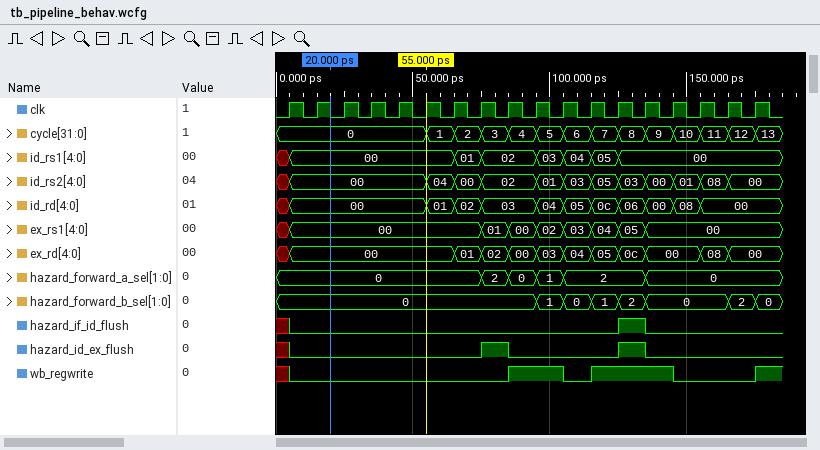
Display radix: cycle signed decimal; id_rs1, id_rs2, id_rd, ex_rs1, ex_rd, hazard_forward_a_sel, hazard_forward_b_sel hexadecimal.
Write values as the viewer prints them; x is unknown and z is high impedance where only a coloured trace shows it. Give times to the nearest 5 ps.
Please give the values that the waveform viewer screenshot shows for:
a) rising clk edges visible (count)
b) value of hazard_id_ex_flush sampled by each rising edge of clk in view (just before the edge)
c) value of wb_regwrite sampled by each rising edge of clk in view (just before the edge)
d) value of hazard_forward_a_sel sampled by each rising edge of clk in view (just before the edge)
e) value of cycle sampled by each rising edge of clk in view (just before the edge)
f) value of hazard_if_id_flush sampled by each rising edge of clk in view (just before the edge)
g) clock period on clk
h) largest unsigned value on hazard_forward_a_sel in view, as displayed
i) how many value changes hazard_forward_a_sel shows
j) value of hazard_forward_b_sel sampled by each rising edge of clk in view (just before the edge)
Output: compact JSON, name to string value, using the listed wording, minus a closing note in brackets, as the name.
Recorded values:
{"rising clk edges visible": "18", "value of hazard_id_ex_flush sampled by each rising edge of clk in view": "x 0 0 0 0 0 0 0 1 0 0 0 0 1 0 0 0 0", "value of wb_regwrite sampled by each rising edge of clk in view": "x 0 0 0 0 0 0 0 0 1 1 0 1 1 1 0 0 0", "value of hazard_forward_a_sel sampled by each rising edge of clk in view": "0, 0, 0, 0, 0, 0, 0, 0, 2, 0, 1, 2, 2, 2, 0, 0, 0, 0", "value of cycle sampled by each rising edge of clk in view": "0, 0, 0, 0, 0, 0, 1, 2, 3, 4, 5, 6, 7, 8, 9, 10, 11, 12", "value of hazard_if_id_flush sampled by each rising edge of clk in view": "x 0 0 0 0 0 0 0 0 0 0 0 0 1 0 0 0 0", "clock period on clk": "10 ps", "largest unsigned value on hazard_forward_a_sel in view, as displayed": "2", "how many value changes hazard_forward_a_sel shows": "5", "value of hazard_forward_b_sel sampled by each rising edge of clk in view": "0, 0, 0, 0, 0, 0, 0, 0, 0, 0, 1, 0, 1, 2, 0, 0, 0, 2"}
